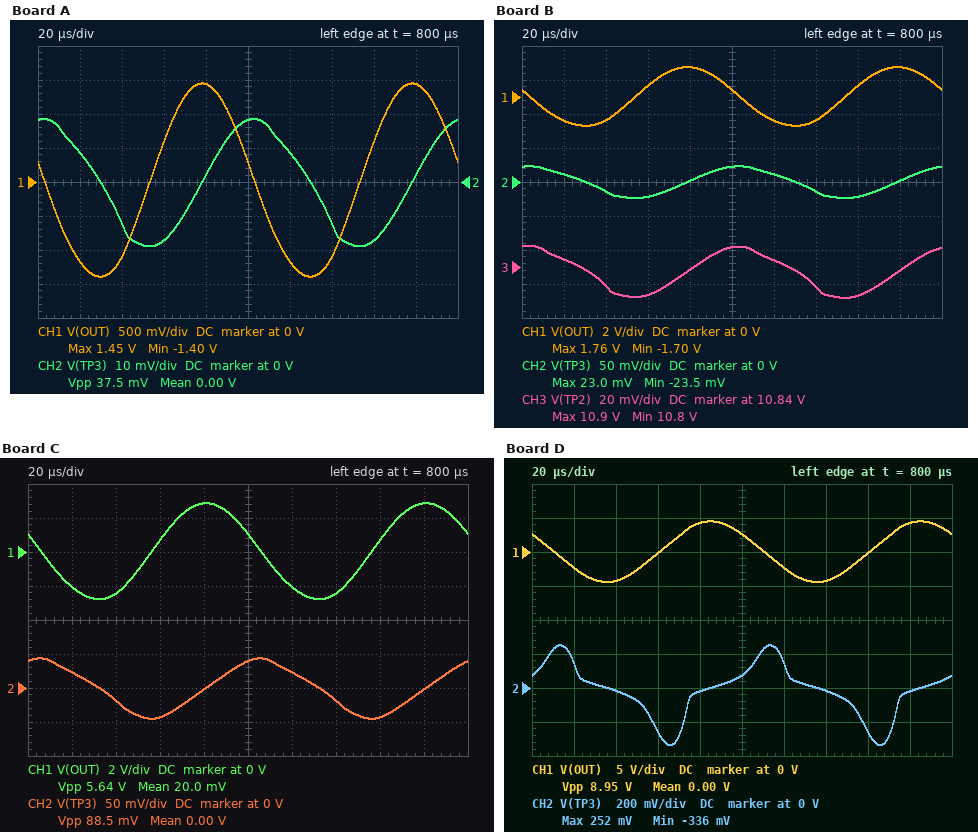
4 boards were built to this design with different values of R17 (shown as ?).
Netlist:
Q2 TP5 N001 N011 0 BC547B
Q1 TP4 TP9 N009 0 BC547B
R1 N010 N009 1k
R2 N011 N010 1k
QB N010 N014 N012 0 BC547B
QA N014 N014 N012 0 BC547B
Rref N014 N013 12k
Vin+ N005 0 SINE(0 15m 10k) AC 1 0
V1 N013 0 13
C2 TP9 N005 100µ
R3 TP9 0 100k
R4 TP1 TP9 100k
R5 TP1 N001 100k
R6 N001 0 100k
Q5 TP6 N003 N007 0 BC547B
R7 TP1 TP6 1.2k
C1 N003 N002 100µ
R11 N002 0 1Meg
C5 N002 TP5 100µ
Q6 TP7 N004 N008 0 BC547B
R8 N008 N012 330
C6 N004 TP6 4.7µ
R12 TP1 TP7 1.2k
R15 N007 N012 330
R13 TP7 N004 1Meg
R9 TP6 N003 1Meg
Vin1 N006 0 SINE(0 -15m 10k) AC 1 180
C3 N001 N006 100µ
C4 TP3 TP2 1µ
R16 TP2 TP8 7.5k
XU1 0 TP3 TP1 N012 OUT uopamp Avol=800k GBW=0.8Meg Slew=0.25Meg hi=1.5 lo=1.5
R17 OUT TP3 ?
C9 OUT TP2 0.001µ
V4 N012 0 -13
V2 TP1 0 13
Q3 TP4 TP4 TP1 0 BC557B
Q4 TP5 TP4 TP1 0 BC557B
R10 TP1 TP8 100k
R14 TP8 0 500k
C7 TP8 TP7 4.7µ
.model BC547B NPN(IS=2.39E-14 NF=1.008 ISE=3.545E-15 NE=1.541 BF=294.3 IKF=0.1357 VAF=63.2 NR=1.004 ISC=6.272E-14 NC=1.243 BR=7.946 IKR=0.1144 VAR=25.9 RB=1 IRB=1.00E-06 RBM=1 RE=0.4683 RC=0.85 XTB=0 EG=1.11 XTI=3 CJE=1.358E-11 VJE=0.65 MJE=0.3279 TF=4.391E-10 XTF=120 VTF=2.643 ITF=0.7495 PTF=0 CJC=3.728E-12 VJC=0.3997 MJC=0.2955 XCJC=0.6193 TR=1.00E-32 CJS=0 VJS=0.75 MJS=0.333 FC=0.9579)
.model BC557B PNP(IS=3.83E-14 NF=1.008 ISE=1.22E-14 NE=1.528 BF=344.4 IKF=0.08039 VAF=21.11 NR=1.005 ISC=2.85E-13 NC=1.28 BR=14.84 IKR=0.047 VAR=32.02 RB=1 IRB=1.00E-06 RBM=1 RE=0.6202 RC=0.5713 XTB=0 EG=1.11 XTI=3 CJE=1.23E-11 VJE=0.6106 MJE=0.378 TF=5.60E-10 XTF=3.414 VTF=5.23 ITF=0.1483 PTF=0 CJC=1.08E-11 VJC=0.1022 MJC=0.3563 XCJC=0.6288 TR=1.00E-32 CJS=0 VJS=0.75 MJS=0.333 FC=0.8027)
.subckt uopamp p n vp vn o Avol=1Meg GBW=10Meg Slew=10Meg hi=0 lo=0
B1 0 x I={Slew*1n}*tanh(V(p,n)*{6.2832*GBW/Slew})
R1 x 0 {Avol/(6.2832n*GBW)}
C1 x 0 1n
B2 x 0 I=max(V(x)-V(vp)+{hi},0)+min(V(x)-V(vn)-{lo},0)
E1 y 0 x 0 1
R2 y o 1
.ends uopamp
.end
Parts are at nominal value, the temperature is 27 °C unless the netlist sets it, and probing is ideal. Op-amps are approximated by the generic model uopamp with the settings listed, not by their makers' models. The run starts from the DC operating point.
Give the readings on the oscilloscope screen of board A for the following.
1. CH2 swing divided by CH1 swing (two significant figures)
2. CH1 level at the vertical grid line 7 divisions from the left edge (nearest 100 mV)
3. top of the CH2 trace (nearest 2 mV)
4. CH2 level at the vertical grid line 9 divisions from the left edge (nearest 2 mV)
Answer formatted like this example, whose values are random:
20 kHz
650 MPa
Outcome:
0.013
-1.1 V
18 mV
2 mV
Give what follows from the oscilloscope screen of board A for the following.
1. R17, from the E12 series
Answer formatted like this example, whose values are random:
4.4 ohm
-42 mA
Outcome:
2.7 kΩ
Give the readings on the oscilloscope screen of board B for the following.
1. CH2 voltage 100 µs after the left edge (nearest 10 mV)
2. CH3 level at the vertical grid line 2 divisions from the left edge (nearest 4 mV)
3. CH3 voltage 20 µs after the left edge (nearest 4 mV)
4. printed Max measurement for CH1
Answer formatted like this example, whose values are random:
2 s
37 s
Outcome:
20 mV
10.828 V
10.844 V
1.76 V
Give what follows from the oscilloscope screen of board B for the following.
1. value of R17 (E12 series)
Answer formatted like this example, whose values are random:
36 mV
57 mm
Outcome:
3.3 kΩ
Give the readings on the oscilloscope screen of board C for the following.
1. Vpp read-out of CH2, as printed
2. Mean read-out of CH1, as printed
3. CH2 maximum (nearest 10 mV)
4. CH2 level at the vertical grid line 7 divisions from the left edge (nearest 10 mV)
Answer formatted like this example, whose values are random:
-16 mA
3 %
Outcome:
88.5 mV
20.0 mV
40 mV
-20 mV
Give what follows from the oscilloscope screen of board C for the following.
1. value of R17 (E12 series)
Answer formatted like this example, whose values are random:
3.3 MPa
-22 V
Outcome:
5.6 kΩ
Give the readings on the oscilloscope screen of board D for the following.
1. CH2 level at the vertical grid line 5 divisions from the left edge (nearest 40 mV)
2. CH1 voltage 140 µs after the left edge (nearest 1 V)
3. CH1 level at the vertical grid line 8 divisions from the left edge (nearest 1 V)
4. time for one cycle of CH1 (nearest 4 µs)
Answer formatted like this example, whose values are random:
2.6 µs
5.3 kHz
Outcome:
80 mV
-4 V
0 V
100 µs
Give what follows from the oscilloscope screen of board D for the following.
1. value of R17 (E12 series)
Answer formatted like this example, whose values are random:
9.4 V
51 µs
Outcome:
10 kΩ
